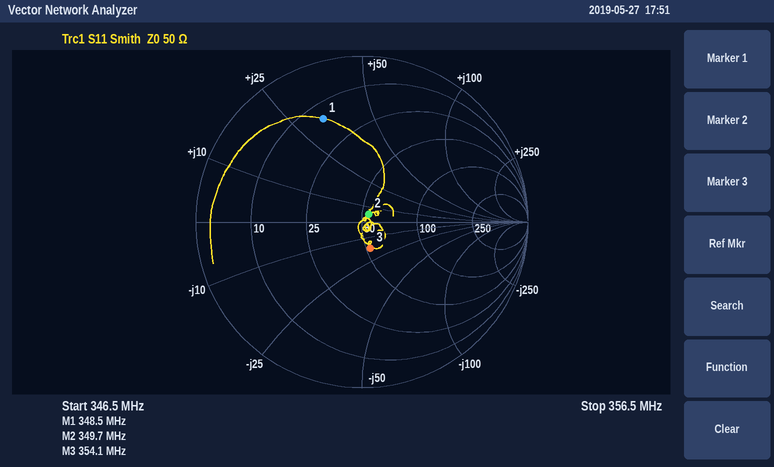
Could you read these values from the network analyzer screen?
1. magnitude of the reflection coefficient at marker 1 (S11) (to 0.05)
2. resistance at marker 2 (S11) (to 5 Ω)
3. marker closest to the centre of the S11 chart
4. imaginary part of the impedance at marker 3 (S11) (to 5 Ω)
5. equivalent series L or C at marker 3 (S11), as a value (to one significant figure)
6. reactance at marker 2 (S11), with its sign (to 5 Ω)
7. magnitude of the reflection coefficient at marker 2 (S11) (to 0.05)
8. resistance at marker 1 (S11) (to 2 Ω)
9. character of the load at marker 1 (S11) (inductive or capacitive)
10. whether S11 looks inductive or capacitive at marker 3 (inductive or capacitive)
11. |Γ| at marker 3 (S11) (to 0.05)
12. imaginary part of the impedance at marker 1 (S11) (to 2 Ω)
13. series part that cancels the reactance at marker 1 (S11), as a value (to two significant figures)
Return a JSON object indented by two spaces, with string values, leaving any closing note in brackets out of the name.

{
  "magnitude of the reflection coefficient at marker 1 (S11)": "0.65",
  "resistance at marker 2 (S11)": "55 Ω",
  "marker closest to the centre of the S11 chart": "marker 2",
  "imaginary part of the impedance at marker 3 (S11)": "-15 Ω",
  "equivalent series L or C at marker 3 (S11), as a value": "30 pF",
  "reactance at marker 2 (S11), with its sign": "+5 Ω",
  "magnitude of the reflection coefficient at marker 2 (S11)": "0.05",
  "resistance at marker 1 (S11)": "14 Ω",
  "character of the load at marker 1 (S11)": "inductive",
  "whether S11 looks inductive or capacitive at marker 3": "capacitive",
  "|Γ| at marker 3 (S11)": "0.15",
  "imaginary part of the impedance at marker 1 (S11)": "+32 Ω",
  "series part that cancels the reactance at marker 1 (S11), as a value": "14 pF"
}
